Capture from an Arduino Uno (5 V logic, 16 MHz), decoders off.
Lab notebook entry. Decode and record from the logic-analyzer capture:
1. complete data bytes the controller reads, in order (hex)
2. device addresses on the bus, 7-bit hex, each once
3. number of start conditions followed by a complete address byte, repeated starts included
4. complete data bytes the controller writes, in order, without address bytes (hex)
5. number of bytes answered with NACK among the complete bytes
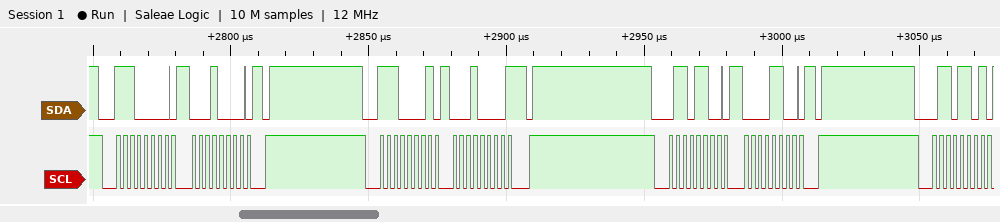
10
0x70 0x36
4
10 0C
1
